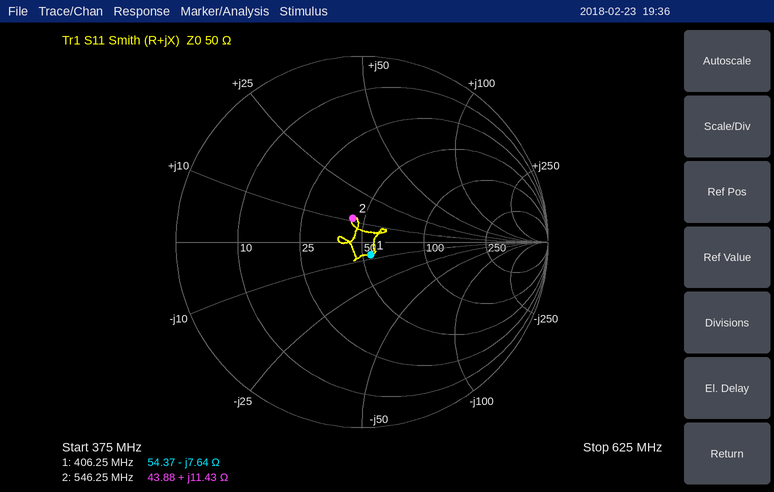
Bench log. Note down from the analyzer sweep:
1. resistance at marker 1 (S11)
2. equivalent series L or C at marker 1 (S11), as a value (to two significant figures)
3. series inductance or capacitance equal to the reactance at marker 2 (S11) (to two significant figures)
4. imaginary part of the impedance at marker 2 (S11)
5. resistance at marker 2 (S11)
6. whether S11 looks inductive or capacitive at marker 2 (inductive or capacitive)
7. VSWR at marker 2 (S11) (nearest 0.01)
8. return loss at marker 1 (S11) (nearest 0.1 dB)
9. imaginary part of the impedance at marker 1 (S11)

54.37 Ω
51 pF
3.3 nH
+11.43 Ω
43.88 Ω
inductive
1.32
21.5 dB
-7.64 Ω
